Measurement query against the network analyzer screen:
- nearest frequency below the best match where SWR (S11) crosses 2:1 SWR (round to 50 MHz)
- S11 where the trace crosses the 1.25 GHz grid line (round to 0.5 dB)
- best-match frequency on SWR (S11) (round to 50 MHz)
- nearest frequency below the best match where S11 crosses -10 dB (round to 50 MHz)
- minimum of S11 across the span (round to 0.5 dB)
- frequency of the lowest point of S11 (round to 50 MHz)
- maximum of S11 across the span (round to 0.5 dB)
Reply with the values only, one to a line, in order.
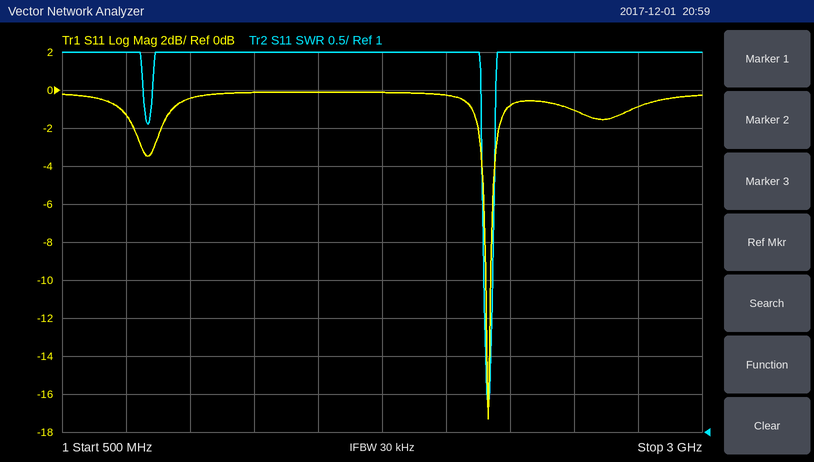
2.15 GHz
0.0 dB
2.15 GHz
2.15 GHz
-17.5 dB
2.15 GHz
0.0 dB
